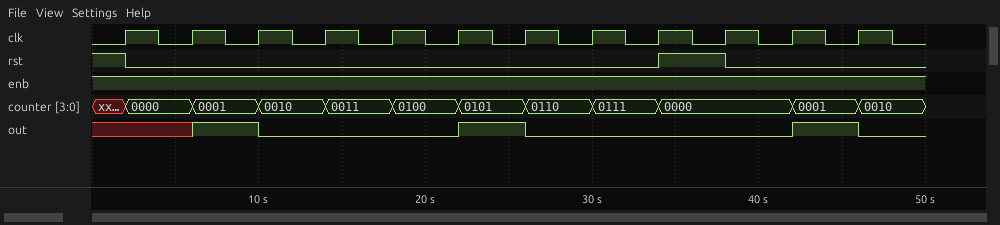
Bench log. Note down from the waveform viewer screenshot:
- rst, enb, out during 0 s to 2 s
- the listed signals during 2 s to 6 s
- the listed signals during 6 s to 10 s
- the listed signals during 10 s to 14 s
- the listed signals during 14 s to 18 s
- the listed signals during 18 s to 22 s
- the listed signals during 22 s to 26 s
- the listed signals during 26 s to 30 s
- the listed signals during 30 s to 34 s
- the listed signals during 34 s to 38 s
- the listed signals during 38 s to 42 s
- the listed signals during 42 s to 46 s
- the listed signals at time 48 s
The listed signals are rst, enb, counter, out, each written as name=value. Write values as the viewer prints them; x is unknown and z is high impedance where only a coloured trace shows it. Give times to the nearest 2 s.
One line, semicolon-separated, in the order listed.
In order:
rst=1, enb=1, out=x; rst=0, enb=1, counter=0000, out=x; rst=0, enb=1, counter=0001, out=1; rst=0, enb=1, counter=0010, out=0; rst=0, enb=1, counter=0011, out=0; rst=0, enb=1, counter=0100, out=0; rst=0, enb=1, counter=0101, out=1; rst=0, enb=1, counter=0110, out=0; rst=0, enb=1, counter=0111, out=0; rst=1, enb=1, counter=0000, out=0; rst=0, enb=1, counter=0000, out=0; rst=0, enb=1, counter=0001, out=1; rst=0, enb=1, counter=0010, out=0
